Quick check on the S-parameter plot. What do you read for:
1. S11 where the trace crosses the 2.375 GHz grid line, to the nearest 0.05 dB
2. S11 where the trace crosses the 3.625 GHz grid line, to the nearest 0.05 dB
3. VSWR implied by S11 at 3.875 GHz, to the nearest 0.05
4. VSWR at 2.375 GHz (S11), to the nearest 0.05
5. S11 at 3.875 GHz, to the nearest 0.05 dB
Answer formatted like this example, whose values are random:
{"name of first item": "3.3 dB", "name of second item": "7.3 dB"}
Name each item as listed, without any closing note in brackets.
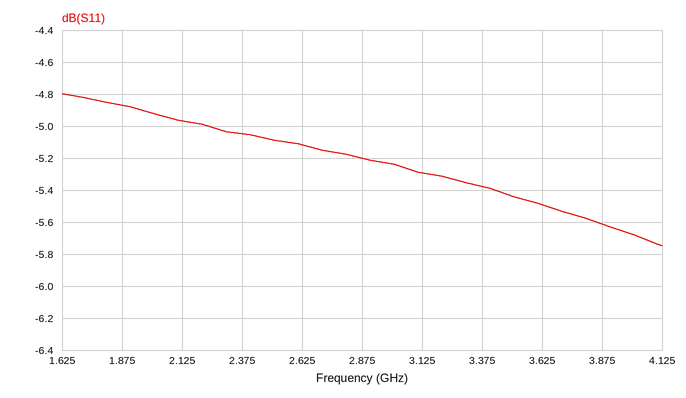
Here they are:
{"S11 where the trace crosses the 2.375 GHz grid line, to the nearest 0.05 dB": "-5.05 dB", "S11 where the trace crosses the 3.625 GHz grid line, to the nearest 0.05 dB": "-5.50 dB", "VSWR implied by S11 at 3.875 GHz, to the nearest 0.05": "3.20", "VSWR at 2.375 GHz (S11), to the nearest 0.05": "3.55", "S11 at 3.875 GHz, to the nearest 0.05 dB": "-5.60 dB"}
